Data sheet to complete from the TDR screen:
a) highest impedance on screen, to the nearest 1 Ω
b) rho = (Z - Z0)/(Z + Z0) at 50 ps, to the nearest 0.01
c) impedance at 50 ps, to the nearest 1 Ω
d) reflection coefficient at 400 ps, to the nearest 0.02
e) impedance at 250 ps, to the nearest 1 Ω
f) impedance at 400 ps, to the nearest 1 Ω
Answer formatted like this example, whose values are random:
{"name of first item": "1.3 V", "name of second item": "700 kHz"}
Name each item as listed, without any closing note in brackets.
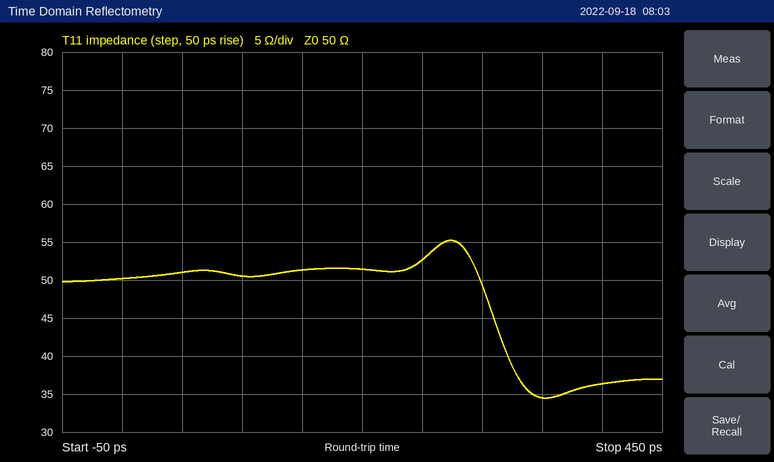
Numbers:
{"highest impedance on screen, to the nearest 1 Ω": "55 Ω", "rho = (Z - Z0)/(Z + Z0) at 50 ps, to the nearest 0.01": "+0.01", "impedance at 50 ps, to the nearest 1 Ω": "51 Ω", "reflection coefficient at 400 ps, to the nearest 0.02": "-0.16", "impedance at 250 ps, to the nearest 1 Ω": "53 Ω", "impedance at 400 ps, to the nearest 1 Ω": "36 Ω"}
